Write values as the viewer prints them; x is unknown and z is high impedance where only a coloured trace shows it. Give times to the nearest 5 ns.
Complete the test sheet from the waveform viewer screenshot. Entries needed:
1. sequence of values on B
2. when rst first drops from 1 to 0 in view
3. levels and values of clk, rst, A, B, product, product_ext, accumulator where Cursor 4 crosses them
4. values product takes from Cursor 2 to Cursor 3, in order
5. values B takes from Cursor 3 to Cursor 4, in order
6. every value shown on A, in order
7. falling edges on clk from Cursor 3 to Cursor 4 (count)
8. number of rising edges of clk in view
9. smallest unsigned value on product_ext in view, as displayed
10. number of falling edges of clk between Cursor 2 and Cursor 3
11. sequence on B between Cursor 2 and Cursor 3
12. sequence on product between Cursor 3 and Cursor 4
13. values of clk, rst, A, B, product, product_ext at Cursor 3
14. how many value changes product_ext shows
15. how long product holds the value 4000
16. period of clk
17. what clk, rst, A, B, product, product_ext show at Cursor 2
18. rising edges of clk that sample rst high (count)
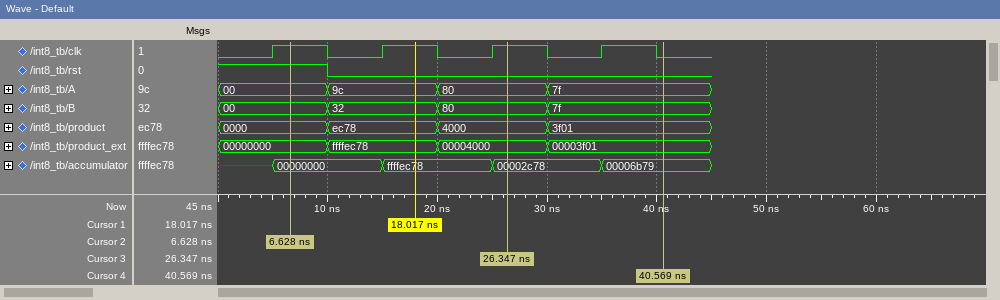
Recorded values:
00, 32, 80, 7f
10 ns
clk=0, rst=0, A=7f, B=7f, product=3f01, product_ext=00003f01, accumulator=00006b79
0000, ec78, 4000
80, 7f
00, 9c, 80, 7f
2
4
00000000
2
00, 32, 80
4000, 3f01
clk=1, rst=0, A=80, B=80, product=4000, product_ext=00004000
3
10 ns
10 ns
clk=1, rst=1, A=00, B=00, product=0000, product_ext=00000000
1
